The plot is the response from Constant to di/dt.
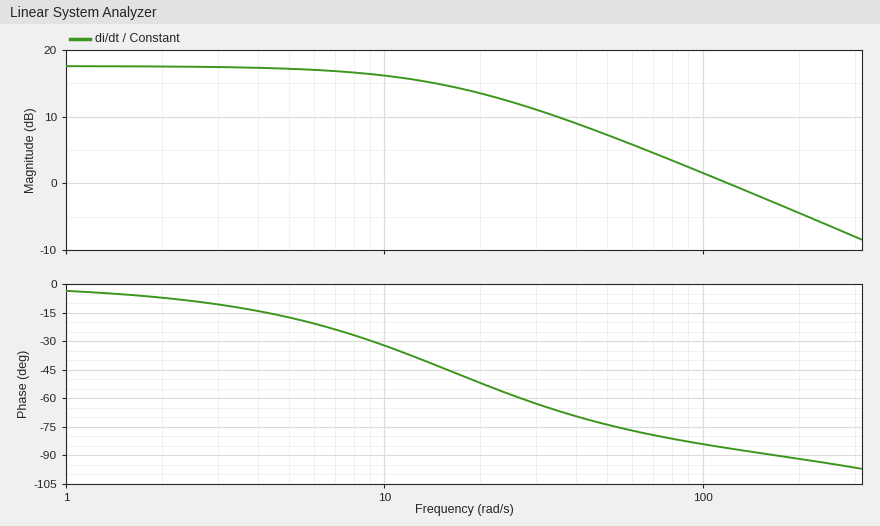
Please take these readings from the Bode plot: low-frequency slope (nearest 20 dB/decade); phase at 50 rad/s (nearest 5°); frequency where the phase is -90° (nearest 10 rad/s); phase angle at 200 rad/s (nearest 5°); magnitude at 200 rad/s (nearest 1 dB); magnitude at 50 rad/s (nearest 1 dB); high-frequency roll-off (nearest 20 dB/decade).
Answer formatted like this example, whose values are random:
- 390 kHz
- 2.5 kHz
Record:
- 0 dB/decade
- -75°
- 170 rad/s
- -90°
- -4 dB
- 7 dB
- -20 dB/decade
